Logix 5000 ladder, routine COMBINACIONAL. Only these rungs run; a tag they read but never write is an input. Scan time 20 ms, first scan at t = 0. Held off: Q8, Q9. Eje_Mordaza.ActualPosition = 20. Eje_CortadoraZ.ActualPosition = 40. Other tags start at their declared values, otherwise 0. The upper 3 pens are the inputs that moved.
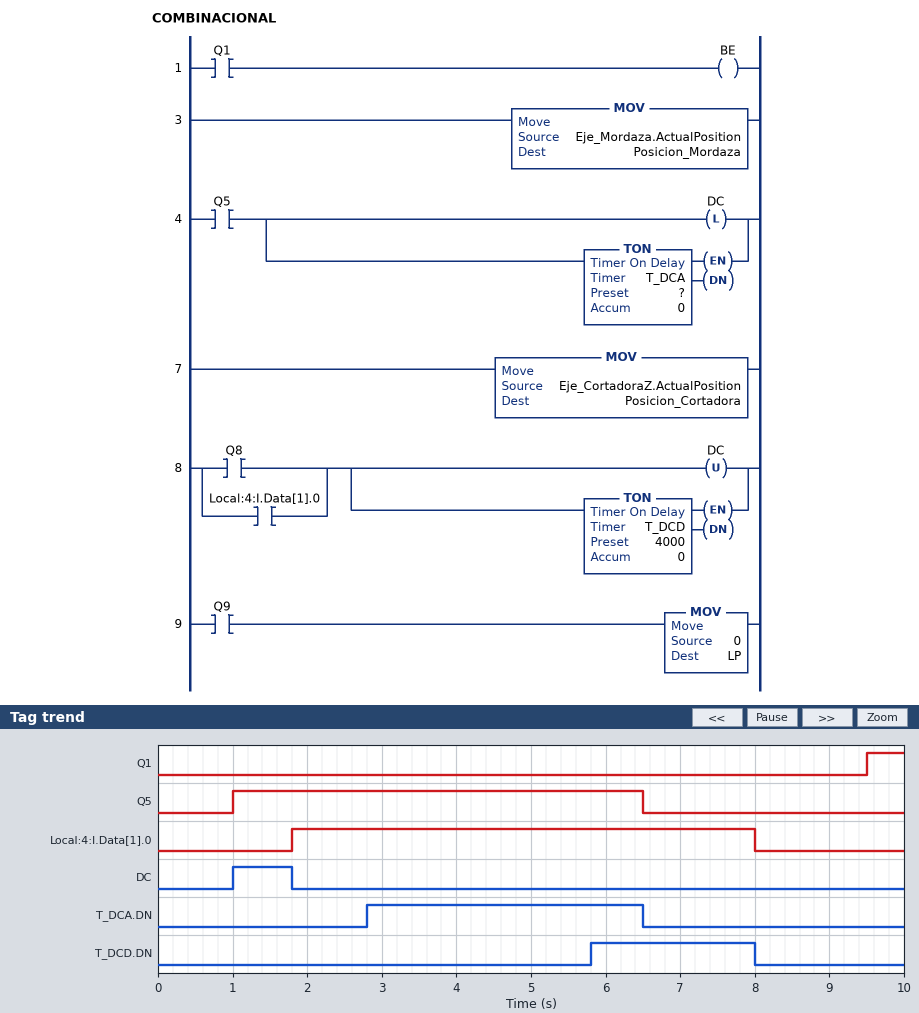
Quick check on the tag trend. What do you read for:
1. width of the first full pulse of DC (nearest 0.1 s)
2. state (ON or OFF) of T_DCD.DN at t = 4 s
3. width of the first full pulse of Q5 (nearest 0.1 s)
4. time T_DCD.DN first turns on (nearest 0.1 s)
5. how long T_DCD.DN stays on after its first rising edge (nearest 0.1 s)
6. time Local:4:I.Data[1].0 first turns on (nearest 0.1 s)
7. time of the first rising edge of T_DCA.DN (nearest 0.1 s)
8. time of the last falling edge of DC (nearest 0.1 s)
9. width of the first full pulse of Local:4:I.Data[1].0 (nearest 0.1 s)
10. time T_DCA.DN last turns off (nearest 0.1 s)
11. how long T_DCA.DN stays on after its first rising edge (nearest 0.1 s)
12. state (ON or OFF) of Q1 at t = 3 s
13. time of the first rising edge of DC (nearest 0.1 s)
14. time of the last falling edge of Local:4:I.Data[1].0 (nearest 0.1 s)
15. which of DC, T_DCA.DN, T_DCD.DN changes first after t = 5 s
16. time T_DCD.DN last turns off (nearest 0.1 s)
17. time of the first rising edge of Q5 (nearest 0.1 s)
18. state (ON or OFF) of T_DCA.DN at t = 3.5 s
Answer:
0.8 s
OFF
5.5 s
5.8 s
2.2 s
1.8 s
2.8 s
1.8 s
6.2 s
6.5 s
3.7 s
OFF
1.0 s
8.0 s
T_DCD.DN
8.0 s
1.0 s
ON
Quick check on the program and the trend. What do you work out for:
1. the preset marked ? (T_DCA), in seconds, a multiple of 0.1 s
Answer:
1.8 s
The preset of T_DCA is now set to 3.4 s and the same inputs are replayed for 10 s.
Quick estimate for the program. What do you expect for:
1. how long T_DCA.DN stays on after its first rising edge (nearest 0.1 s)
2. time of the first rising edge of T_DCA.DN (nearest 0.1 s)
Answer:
2.1 s
4.4 s
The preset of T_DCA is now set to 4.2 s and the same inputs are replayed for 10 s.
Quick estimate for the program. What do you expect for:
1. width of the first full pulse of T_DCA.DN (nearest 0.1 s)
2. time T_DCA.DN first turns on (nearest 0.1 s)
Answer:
1.3 s
5.2 s
